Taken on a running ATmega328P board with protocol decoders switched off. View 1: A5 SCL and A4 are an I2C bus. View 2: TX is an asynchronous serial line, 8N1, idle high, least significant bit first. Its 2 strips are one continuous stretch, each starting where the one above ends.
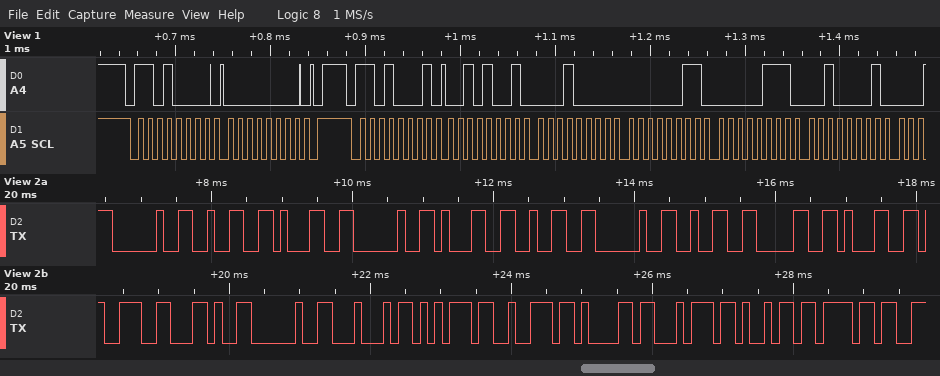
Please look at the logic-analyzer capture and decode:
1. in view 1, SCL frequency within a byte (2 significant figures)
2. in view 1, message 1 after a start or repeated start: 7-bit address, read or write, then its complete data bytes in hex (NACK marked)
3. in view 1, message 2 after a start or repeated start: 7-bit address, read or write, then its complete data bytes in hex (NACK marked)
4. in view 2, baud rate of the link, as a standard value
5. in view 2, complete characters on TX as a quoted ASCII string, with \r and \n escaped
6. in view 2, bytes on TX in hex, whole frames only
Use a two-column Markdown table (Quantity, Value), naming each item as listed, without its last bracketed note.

| Quantity | Value |
|---|---|
| in view 1, SCL frequency within a byte | 100 kHz |
| in view 1, message 1 after a start or repeated start: 7-bit address, read or write, then its complete data bytes in hex | 0x68 write: 00 |
| in view 1, message 2 after a start or repeated start: 7-bit address, read or write, then its complete data bytes in hex | 0x68 read: 29 10 03 07 21 |
| in view 2, baud rate of the link, as a standard value | 9600 baud |
| in view 2, complete characters on TX as a quoted ASCII string, with \r and \n escaped | " 21 12 2019, Duratio" |
| in view 2, bytes on TX in hex, whole frames only | 0x20 0x32 0x31 0x20 0x31 0x32 0x20 0x32 0x30 0x31 0x39 0x2C 0x20 0x44 0x75 0x72 0x61 0x74 0x69 0x6F |
